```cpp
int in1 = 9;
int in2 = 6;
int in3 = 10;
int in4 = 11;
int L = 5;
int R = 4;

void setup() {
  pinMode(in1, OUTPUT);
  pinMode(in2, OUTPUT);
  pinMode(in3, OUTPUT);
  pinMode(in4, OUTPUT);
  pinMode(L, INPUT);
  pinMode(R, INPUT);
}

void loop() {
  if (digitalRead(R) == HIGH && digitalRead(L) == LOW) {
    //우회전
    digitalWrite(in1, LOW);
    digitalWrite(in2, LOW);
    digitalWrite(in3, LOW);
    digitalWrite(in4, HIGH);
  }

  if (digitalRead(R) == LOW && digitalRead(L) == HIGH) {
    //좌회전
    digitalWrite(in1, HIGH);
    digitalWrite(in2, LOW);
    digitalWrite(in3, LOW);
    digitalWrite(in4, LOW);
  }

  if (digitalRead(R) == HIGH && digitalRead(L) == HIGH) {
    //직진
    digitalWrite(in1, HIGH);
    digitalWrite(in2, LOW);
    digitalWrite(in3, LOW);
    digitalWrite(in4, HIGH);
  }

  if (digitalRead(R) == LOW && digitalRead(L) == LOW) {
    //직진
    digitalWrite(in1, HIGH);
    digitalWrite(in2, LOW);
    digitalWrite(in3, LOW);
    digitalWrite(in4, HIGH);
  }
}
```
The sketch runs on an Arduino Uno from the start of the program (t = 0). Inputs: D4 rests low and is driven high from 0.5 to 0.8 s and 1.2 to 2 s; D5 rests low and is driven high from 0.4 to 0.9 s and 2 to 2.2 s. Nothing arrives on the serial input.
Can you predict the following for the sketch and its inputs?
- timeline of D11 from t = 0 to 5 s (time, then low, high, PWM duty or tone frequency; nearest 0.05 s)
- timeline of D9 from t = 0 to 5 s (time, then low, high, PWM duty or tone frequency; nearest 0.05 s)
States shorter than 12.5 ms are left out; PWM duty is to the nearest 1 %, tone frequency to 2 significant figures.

0 s high; 0.4 s low; 0.5 s high; 0.8 s low; 0.9 s high; 2 s low; 2.2 s high
0 s high; 1.2 s low; 2 s high
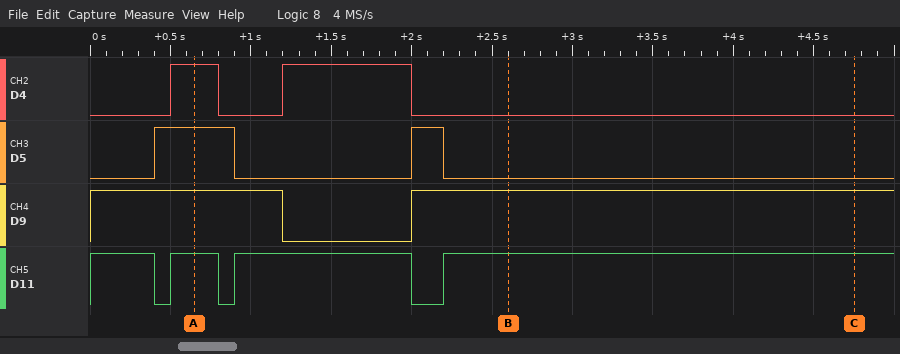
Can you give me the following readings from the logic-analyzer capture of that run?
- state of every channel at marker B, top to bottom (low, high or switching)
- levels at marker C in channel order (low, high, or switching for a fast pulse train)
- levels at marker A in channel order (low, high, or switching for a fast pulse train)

D4 low, D5 low, D9 high, D11 high
D4 low, D5 low, D9 high, D11 high
D4 high, D5 high, D9 high, D11 high
